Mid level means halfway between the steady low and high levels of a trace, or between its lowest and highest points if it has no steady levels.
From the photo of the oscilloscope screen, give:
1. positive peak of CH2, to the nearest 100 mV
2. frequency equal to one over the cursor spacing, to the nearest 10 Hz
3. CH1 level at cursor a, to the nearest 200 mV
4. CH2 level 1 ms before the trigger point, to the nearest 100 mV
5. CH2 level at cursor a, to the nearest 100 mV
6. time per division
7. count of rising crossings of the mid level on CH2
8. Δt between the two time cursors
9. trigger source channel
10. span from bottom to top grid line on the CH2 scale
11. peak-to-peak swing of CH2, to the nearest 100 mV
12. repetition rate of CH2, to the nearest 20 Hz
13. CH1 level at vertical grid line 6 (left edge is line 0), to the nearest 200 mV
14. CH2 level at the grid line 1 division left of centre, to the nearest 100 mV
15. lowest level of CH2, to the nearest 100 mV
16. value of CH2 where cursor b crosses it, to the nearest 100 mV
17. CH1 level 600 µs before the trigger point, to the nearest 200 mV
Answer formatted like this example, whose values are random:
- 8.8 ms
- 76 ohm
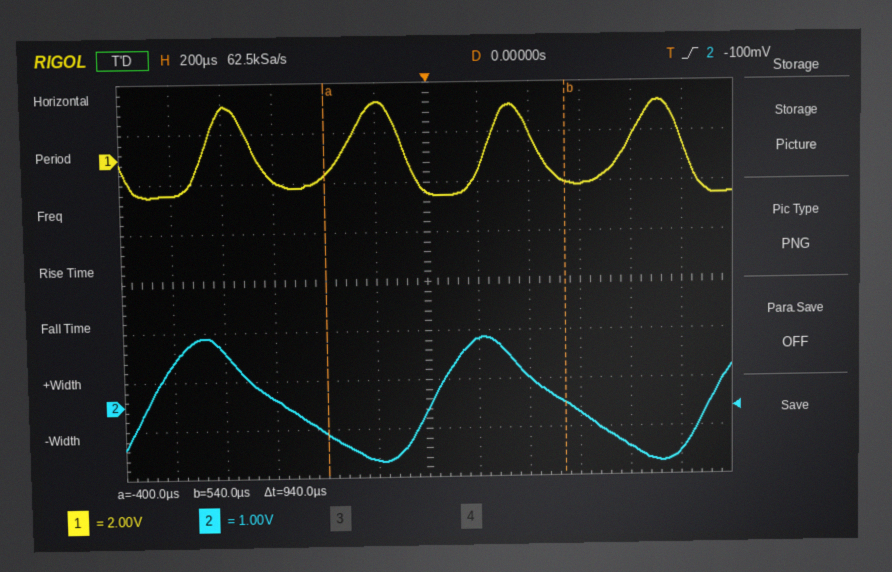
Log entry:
- 1.4 V
- 1.06 kHz
- -600 mV
- 900 mV
- -600 mV
- 200 µs
- 3
- 940 µs
- CH2
- 8 V
- 2.6 V
- 900 Hz
- -1.4 V
- -1.1 V
- -1.2 V
- 0.0 V
- -800 mV
